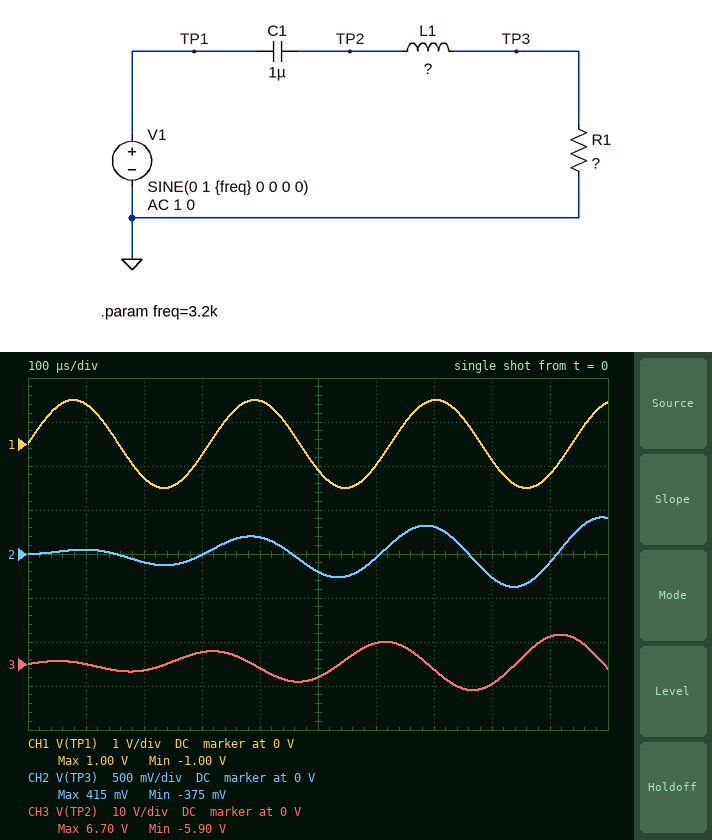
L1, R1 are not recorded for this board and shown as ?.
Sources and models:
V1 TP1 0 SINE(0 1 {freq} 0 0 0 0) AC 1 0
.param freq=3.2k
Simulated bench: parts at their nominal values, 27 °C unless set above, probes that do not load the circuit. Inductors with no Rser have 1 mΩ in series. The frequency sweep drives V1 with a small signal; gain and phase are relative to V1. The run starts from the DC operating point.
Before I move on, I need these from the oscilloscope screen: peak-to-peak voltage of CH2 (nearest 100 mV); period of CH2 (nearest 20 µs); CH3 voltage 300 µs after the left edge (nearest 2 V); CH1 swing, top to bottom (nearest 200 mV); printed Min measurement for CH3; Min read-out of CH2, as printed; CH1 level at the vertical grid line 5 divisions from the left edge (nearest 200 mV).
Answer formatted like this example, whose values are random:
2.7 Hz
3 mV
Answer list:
800 mV
300 µs
2 V
2.0 V
-5.90 V
-375 mV
-600 mV
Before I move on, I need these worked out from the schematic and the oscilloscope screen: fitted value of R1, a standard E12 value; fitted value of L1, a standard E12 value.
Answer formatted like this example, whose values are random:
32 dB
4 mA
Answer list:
2.7 Ω
2.2 mH
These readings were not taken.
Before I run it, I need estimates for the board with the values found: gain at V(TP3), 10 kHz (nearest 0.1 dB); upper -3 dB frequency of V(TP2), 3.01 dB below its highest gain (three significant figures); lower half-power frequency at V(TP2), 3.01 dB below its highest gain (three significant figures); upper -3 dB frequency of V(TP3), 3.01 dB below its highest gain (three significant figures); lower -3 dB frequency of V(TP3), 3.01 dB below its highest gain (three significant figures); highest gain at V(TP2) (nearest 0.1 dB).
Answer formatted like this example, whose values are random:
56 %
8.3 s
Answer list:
-33.1 dB
3.50 kHz
3.30 kHz
3.49 kHz
3.30 kHz
24.8 dB
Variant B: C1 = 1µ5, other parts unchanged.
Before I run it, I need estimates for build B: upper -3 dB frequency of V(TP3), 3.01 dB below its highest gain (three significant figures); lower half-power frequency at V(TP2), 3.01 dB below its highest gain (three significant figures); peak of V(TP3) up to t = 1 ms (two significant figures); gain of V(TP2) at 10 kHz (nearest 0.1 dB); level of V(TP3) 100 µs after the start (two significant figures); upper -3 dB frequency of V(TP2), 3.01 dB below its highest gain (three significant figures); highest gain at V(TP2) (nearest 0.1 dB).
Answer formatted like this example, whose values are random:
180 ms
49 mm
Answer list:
2.87 kHz
2.68 kHz
330 mV
0.7 dB
60 mV
2.88 kHz
23.1 dB
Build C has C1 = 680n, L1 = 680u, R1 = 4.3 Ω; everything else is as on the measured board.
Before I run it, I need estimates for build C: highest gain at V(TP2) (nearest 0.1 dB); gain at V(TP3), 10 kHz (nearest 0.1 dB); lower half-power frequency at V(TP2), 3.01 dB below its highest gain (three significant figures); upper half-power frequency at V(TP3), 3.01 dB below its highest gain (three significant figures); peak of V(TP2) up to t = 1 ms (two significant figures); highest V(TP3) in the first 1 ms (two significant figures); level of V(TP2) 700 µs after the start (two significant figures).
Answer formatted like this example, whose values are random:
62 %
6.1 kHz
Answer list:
17.4 dB
-13.3 dB
6.97 kHz
7.92 kHz
400 mV
92 mV
-170 mV
